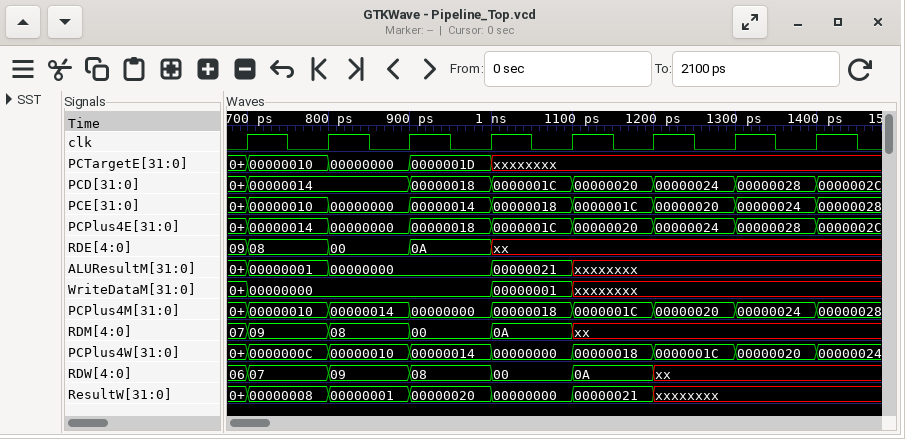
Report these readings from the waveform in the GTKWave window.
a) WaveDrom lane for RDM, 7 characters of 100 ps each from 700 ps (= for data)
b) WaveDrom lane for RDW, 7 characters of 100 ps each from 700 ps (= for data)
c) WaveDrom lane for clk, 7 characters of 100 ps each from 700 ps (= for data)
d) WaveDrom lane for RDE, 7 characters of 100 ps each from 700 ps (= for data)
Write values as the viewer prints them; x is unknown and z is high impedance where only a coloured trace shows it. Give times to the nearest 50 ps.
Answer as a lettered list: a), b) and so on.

a) {name: 'RDM', wave: '====x..', data: '09 08 00 0A'}
b) {name: 'RDW', wave: '=====x.', data: '07 09 08 00 0A'}
c) {name: 'clk', wave: 'p......'}
d) {name: 'RDE', wave: '===x...', data: '08 00 0A'}
